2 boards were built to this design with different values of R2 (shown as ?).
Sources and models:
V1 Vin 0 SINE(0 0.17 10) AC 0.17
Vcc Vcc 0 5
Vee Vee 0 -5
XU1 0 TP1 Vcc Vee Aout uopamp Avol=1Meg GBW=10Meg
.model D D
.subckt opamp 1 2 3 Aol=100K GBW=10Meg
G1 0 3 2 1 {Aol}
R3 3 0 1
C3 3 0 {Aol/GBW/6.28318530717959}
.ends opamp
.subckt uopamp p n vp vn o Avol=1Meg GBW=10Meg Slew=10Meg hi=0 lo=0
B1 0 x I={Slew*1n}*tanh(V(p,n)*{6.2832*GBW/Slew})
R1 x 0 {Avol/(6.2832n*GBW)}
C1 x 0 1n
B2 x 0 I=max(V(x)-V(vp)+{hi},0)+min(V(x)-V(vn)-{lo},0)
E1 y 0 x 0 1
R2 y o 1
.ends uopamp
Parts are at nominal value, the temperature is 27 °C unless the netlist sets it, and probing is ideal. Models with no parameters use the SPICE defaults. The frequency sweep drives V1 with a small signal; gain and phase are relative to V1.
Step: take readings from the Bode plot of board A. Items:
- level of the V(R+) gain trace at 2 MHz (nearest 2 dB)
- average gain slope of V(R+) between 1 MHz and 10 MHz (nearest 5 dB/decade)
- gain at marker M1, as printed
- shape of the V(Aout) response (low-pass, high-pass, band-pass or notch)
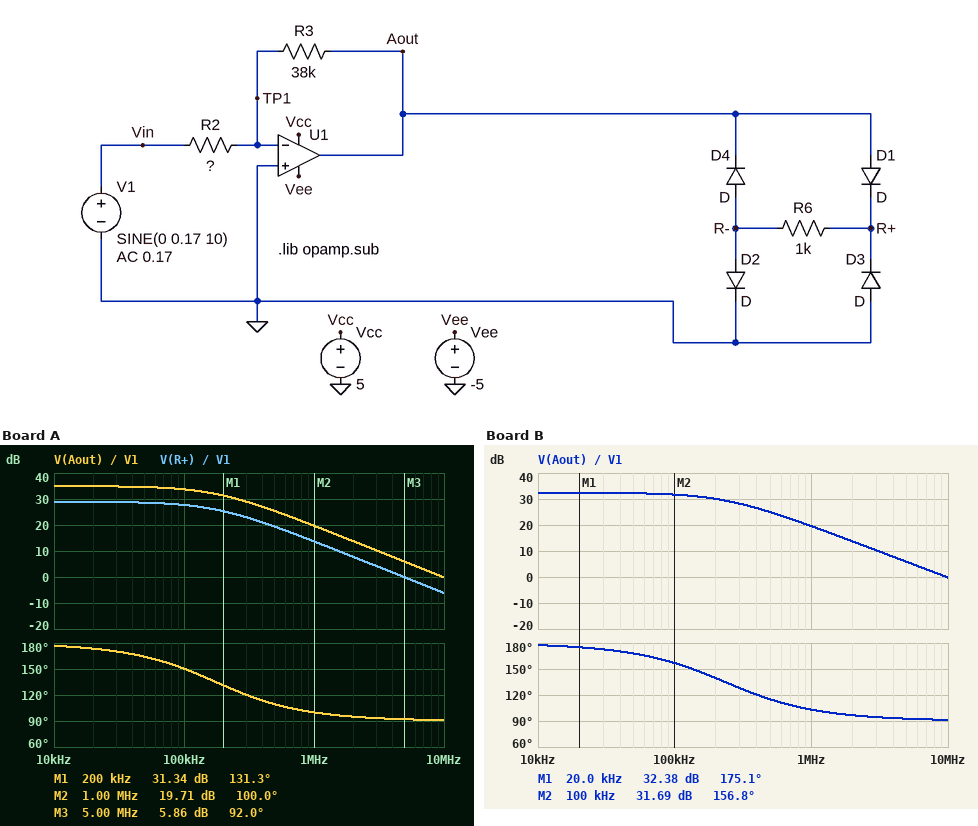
8 dB
-20 dB/decade
31.34 dB
low-pass
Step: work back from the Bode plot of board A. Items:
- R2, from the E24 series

680 Ω
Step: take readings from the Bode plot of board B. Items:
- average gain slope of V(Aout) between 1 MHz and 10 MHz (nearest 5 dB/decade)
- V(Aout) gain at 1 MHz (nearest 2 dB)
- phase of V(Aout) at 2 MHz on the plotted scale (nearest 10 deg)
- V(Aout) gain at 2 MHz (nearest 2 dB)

-20 dB/decade
20 dB
100 deg
14 dB
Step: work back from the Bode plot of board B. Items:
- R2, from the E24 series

910 Ω
